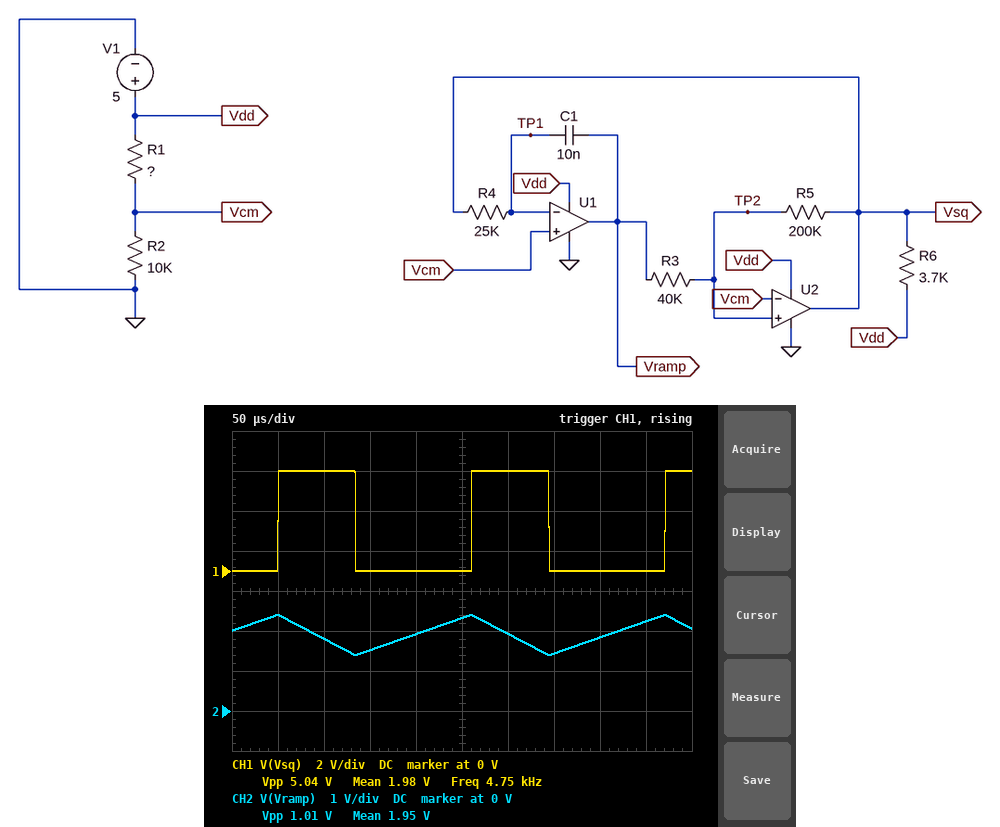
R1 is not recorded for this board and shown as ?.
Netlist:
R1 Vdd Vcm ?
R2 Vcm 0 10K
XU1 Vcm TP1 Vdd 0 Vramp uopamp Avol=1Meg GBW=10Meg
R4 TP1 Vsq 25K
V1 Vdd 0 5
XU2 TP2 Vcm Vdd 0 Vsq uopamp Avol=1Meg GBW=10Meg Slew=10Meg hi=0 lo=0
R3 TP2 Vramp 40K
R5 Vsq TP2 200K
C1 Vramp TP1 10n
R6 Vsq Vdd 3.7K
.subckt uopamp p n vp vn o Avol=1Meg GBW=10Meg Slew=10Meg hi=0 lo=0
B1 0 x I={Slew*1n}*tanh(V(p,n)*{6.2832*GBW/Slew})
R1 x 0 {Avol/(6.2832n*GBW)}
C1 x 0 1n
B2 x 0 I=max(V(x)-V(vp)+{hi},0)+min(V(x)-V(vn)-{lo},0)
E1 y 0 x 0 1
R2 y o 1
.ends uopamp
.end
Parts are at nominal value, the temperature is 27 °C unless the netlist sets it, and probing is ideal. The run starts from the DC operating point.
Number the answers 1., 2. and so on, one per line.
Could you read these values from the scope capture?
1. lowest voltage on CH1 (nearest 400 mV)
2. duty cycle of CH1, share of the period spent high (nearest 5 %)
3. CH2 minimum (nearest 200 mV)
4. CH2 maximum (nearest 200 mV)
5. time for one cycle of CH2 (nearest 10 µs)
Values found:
1. 0 V
2. 40 %
3. 1.4 V
4. 2.4 V
5. 210 µs
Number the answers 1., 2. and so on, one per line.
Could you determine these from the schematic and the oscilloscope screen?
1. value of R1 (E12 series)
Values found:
1. 15 kΩ
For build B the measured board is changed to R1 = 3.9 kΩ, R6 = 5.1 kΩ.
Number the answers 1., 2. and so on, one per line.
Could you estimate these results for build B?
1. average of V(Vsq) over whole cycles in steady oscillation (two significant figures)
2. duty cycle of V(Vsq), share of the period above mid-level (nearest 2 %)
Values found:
1. 3.6 V
2. 72 %
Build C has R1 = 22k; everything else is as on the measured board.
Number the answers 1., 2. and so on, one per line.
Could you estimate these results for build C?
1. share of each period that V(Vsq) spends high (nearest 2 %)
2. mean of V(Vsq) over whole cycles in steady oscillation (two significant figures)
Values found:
1. 32 %
2. 1.6 V
